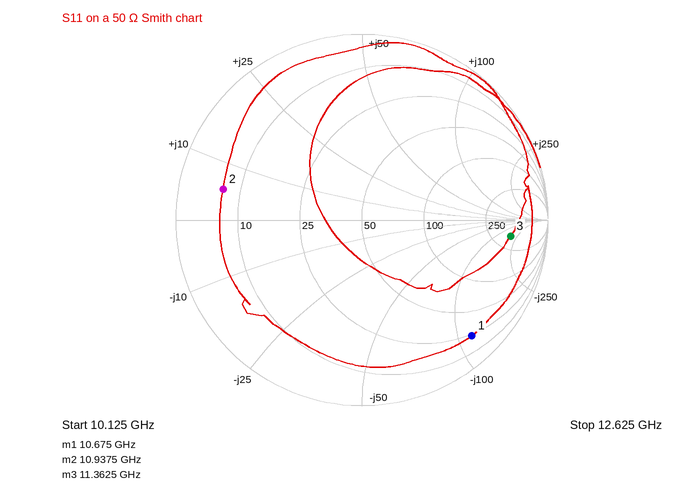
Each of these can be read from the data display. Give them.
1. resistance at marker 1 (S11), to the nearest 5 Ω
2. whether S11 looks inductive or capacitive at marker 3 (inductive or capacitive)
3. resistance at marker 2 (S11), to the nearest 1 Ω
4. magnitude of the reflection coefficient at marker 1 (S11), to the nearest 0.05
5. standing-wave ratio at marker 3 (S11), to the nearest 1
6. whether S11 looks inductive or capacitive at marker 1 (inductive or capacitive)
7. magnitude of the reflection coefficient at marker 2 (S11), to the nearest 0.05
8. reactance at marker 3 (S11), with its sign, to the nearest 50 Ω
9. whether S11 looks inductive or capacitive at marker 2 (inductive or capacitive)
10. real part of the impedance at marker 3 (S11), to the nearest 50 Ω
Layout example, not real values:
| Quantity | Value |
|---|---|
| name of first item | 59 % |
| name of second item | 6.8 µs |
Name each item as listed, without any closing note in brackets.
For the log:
| Quantity | Value |
|---|---|
| resistance at marker 1 (S11), to the nearest 5 Ω | 25 Ω |
| whether S11 looks inductive or capacitive at marker 3 | capacitive |
| resistance at marker 2 (S11), to the nearest 1 Ω | 7 Ω |
| magnitude of the reflection coefficient at marker 1 (S11), to the nearest 0.05 | 0.85 |
| standing-wave ratio at marker 3 (S11), to the nearest 1 | 9 |
| whether S11 looks inductive or capacitive at marker 1 | capacitive |
| magnitude of the reflection coefficient at marker 2 (S11), to the nearest 0.05 | 0.75 |
| reactance at marker 3 (S11), with its sign, to the nearest 50 Ω | -200 Ω |
| whether S11 looks inductive or capacitive at marker 2 | inductive |
| real part of the impedance at marker 3 (S11), to the nearest 50 Ω | 350 Ω |
